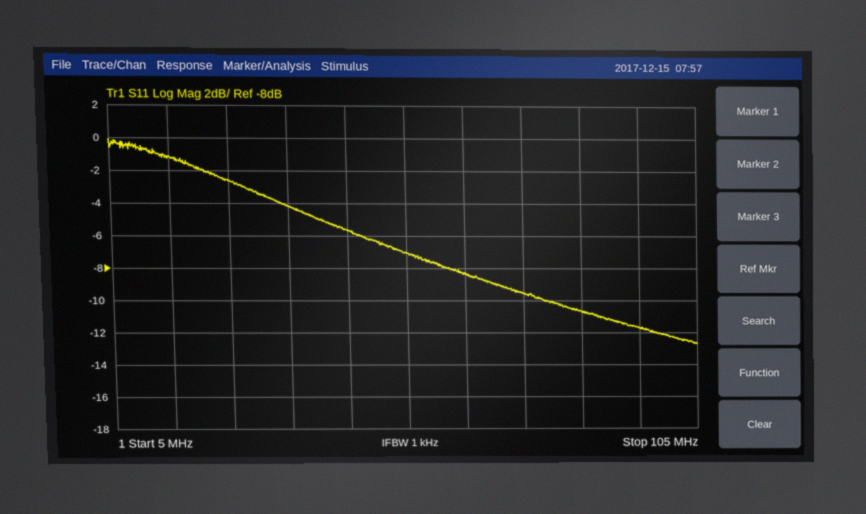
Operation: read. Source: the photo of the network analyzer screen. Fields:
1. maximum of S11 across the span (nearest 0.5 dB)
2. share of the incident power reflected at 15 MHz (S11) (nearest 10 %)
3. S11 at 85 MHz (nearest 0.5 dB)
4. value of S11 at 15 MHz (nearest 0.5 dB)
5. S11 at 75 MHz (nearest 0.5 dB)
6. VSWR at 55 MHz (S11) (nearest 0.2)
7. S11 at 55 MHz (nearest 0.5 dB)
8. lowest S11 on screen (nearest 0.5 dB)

0.0 dB
80 %
-10.5 dB
-1.0 dB
-9.5 dB
2.6
-7.0 dB
-12.5 dB
